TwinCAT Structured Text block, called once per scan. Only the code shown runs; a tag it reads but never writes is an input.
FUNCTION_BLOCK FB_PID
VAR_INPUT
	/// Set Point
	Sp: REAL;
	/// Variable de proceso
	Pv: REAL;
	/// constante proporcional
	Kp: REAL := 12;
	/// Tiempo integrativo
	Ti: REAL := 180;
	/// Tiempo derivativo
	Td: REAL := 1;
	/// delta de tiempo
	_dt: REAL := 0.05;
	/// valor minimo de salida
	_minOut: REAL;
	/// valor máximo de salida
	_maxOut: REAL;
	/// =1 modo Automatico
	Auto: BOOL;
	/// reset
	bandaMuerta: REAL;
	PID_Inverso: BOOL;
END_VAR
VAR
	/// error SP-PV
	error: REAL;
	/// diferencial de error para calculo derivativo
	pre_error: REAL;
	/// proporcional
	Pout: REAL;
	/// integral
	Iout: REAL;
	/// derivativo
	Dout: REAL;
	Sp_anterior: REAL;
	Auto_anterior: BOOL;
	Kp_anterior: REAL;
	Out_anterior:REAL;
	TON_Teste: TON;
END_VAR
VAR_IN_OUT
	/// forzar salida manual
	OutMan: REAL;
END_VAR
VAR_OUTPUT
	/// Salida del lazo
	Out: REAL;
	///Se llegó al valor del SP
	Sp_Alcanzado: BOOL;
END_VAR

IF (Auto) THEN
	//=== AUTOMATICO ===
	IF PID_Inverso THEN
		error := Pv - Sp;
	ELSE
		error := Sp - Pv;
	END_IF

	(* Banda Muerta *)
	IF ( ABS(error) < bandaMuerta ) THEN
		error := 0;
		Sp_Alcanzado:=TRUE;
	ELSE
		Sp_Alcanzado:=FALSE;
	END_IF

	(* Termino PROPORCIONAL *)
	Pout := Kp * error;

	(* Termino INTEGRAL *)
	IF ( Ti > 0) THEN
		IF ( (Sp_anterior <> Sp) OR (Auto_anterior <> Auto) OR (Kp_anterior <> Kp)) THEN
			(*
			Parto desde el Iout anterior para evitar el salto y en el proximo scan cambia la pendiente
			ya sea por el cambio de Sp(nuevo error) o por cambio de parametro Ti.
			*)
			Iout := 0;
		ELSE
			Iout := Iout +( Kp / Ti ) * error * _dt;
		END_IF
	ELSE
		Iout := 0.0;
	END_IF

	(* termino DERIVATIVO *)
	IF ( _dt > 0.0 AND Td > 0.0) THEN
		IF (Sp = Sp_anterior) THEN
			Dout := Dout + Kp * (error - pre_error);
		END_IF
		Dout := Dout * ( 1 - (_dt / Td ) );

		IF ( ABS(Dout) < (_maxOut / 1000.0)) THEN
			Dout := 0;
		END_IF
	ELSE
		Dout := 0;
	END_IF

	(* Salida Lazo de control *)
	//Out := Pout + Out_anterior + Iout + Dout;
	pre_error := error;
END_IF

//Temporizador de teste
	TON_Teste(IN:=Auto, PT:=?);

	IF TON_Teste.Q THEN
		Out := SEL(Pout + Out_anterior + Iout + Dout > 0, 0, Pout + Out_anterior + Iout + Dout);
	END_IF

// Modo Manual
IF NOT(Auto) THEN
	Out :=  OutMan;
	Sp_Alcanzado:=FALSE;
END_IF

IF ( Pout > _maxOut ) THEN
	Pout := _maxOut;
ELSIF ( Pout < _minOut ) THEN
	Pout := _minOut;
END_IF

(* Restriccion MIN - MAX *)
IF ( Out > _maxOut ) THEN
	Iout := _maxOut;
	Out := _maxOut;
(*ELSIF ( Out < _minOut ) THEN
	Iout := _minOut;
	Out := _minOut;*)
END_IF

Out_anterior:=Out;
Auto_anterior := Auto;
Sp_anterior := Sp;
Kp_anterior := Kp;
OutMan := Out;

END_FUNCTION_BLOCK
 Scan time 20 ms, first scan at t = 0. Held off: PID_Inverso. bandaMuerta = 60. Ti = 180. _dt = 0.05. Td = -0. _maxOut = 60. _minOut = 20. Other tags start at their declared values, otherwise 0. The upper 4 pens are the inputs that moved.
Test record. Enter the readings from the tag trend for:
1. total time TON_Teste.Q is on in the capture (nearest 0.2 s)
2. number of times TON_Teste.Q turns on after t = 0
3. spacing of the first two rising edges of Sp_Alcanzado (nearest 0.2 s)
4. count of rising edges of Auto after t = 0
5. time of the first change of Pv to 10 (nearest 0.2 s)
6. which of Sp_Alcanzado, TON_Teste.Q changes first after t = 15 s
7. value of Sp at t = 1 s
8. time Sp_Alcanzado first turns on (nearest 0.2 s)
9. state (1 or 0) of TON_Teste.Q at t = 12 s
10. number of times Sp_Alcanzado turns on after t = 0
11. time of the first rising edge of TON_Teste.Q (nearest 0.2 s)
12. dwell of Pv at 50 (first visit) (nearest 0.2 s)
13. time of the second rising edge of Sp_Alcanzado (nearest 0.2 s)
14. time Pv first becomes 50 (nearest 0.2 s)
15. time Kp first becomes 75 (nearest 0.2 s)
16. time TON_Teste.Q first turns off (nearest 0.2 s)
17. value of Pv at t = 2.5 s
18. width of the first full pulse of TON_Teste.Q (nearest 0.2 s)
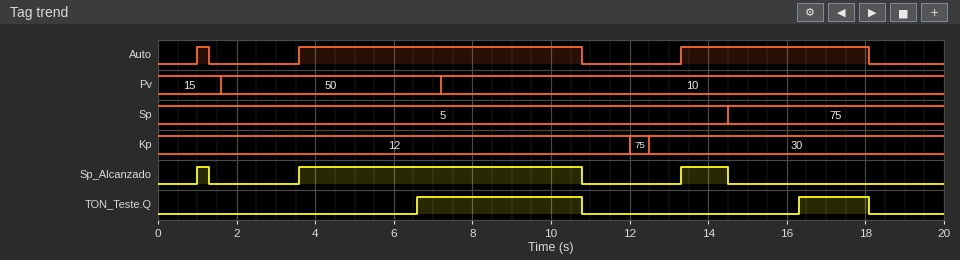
6.0 s
2
2.6 s
3
7.2 s
TON_Teste.Q
5
1.0 s
0
3
6.6 s
5.6 s
3.6 s
1.6 s
12.0 s
10.8 s
50
4.2 s
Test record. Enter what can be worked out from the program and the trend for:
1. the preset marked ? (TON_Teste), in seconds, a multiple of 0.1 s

3.0 s
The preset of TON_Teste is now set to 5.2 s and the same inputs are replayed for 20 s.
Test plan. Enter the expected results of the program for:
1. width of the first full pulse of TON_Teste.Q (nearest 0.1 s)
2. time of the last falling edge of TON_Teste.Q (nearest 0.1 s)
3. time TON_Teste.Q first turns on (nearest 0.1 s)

2.0 s
10.8 s
8.8 s
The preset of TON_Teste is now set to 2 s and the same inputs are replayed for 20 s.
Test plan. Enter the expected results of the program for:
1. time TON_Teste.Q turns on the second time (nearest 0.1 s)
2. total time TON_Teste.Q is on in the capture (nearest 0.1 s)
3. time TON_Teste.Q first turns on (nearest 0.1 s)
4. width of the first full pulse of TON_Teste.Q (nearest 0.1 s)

15.3 s
8.0 s
5.6 s
5.2 s
